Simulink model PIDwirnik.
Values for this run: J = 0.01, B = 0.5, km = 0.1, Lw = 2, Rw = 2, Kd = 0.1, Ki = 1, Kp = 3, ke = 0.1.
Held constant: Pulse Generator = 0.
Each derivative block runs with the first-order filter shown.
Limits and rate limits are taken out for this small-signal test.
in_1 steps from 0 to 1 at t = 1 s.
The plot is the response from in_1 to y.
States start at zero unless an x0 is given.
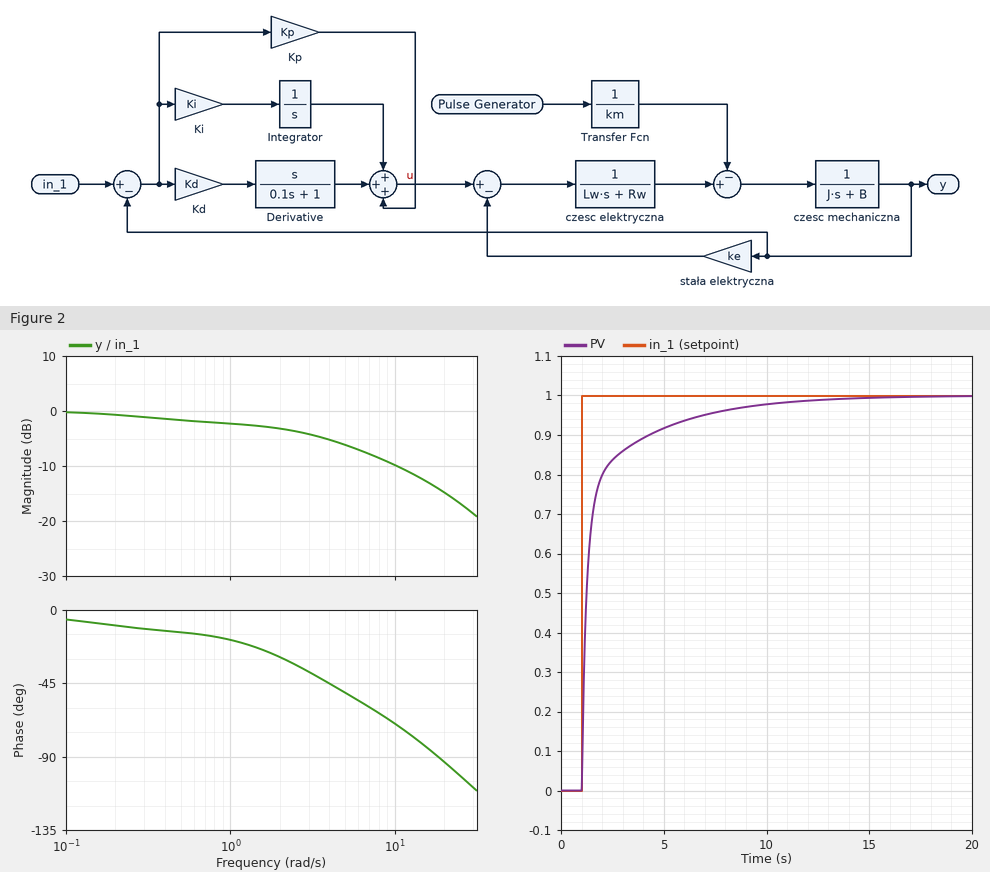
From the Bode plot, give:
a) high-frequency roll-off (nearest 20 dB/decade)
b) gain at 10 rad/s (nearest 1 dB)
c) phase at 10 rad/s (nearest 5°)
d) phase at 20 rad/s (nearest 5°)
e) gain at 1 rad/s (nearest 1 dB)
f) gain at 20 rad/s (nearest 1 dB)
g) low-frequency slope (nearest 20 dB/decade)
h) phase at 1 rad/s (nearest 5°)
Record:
-20 dB/decade
-10 dB
-70°
-95°
-2 dB
-15 dB
0 dB/decade
-20°
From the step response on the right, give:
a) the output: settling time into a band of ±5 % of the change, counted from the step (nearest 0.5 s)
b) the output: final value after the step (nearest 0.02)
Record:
6.0 s
1.00
